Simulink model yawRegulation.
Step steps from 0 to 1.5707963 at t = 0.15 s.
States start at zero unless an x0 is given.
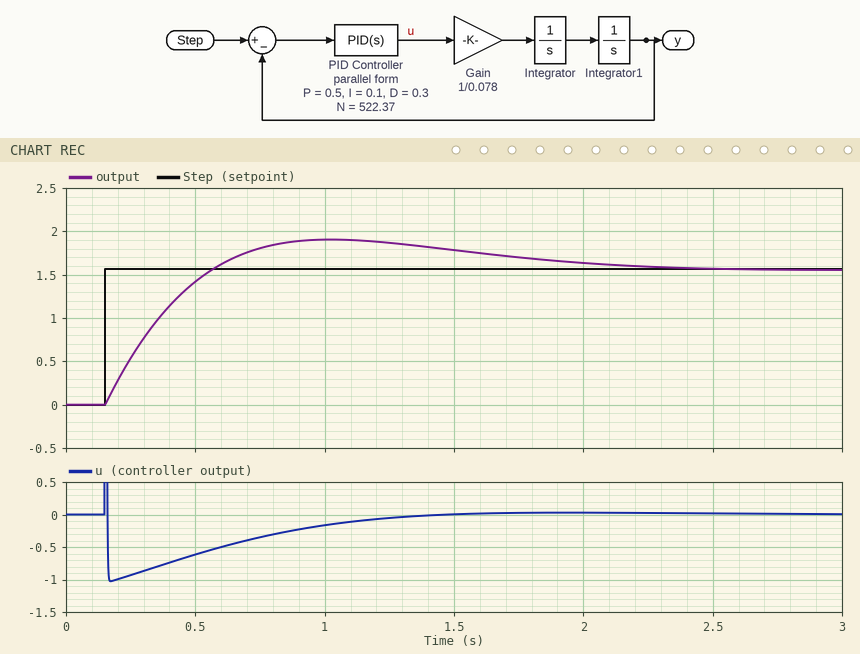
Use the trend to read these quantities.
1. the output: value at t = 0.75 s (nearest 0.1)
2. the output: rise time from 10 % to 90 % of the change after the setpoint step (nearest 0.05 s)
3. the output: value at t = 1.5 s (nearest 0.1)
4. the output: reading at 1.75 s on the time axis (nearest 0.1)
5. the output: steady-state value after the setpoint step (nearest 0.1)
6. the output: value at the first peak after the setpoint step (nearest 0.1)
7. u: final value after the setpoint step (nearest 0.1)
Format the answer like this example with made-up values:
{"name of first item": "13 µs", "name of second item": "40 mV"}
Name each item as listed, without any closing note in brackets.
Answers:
{"the output: value at t = 0.75 s": "1.8", "the output: rise time from 10 % to 90 % of the change after the setpoint step": "0.30 s", "the output: value at t = 1.5 s": "1.8", "the output: reading at 1.75 s on the time axis": "1.7", "the output: steady-state value after the setpoint step": "1.6", "the output: value at the first peak after the setpoint step": "1.9", "u: final value after the setpoint step": "0.0"}
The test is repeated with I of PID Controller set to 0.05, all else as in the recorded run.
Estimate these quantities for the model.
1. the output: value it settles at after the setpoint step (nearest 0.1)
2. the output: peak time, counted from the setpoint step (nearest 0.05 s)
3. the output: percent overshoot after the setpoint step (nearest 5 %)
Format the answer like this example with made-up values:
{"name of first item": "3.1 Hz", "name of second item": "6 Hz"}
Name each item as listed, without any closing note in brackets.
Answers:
{"the output: value it settles at after the setpoint step": "1.6", "the output: peak time, counted from the setpoint step": "0.85 s", "the output: percent overshoot after the setpoint step": "20 %"}
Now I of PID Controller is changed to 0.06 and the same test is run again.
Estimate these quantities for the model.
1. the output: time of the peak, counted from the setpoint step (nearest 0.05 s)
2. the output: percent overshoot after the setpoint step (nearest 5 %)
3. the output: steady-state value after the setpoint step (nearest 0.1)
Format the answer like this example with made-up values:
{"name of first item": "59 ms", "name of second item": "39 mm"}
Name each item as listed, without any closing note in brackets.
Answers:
{"the output: time of the peak, counted from the setpoint step": "0.85 s", "the output: percent overshoot after the setpoint step": "20 %", "the output: steady-state value after the setpoint step": "1.6"}
